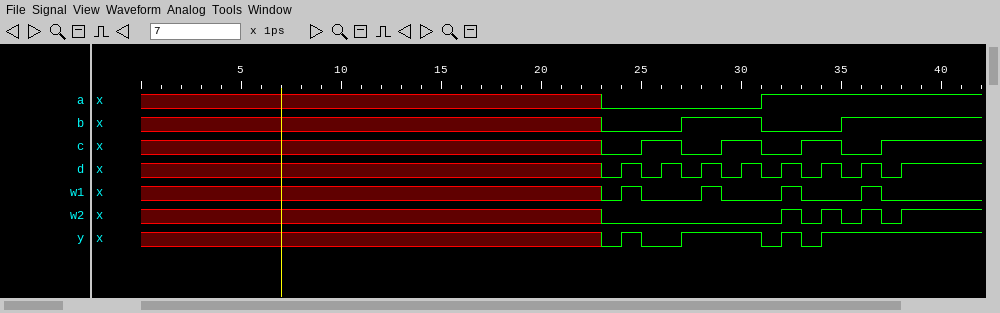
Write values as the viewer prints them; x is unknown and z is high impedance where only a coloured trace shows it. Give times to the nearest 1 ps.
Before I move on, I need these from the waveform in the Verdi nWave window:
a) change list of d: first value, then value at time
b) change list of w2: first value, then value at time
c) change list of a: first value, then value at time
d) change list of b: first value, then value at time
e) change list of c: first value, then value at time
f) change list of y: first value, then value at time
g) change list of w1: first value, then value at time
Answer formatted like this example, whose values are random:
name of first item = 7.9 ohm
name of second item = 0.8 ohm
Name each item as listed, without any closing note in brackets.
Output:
change list of d: first value, then value at time = x, 0 at 23 ps, 1 at 24 ps, 0 at 25 ps, 1 at 26 ps, 0 at 27 ps, 1 at 28 ps, 0 at 29 ps, 1 at 30 ps, 0 at 31 ps, 1 at 32 ps, 0 at 33 ps, 1 at 34 ps, 0 at 35 ps, 1 at 36 ps, 0 at 37 ps, 1 at 38 ps
change list of w2: first value, then value at time = x, 0 at 23 ps, 1 at 32 ps, 0 at 33 ps, 1 at 34 ps, 0 at 35 ps, 1 at 36 ps, 0 at 37 ps, 1 at 38 ps
change list of a: first value, then value at time = x, 0 at 23 ps, 1 at 31 ps
change list of b: first value, then value at time = x, 0 at 23 ps, 1 at 27 ps, 0 at 31 ps, 1 at 35 ps
change list of c: first value, then value at time = x, 0 at 23 ps, 1 at 25 ps, 0 at 27 ps, 1 at 29 ps, 0 at 31 ps, 1 at 33 ps, 0 at 35 ps, 1 at 37 ps
change list of y: first value, then value at time = x, 0 at 23 ps, 1 at 24 ps, 0 at 25 ps, 1 at 27 ps, 0 at 31 ps, 1 at 32 ps, 0 at 33 ps, 1 at 34 ps
change list of w1: first value, then value at time = x, 0 at 23 ps, 1 at 24 ps, 0 at 25 ps, 1 at 28 ps, 0 at 29 ps, 1 at 32 ps, 0 at 33 ps, 1 at 36 ps, 0 at 37 ps
